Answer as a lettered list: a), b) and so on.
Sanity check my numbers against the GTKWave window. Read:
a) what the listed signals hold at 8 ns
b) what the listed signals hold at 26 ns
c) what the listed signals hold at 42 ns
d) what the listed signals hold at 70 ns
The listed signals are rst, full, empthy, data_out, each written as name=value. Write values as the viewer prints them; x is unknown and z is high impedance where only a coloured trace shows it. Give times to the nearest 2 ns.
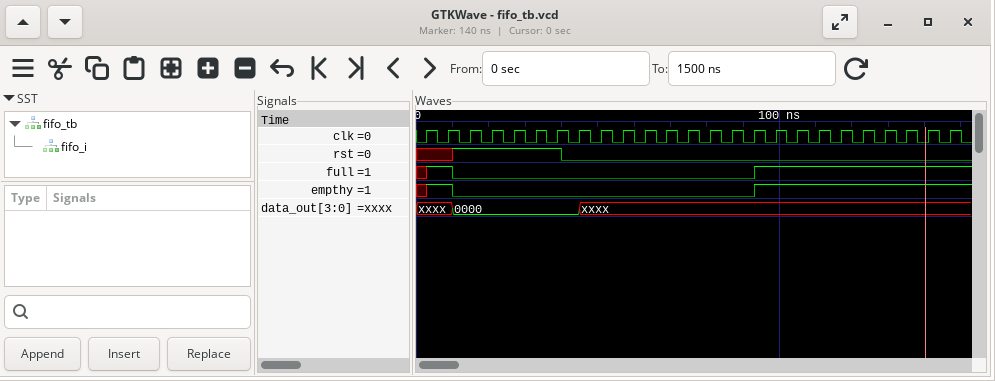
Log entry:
a) rst=x, full=1, empthy=1, data_out=xxxx
b) rst=1, full=0, empthy=0, data_out=0000
c) rst=0, full=0, empthy=0, data_out=0000
d) rst=0, full=0, empthy=0, data_out=xxxx
